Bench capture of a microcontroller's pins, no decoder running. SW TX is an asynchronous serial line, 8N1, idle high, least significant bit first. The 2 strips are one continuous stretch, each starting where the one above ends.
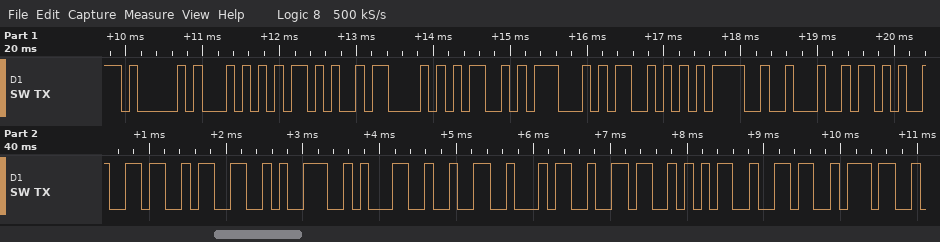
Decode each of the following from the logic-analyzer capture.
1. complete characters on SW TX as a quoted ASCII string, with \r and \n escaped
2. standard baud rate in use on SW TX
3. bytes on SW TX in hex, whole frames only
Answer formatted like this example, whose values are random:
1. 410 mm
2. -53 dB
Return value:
1. "AT+CMGS=\"+6391246567"
2. 9600 baud
3. 41 54 2B 43 4D 47 53 3D 22 2B 36 33 39 31 32 34 36 35 36 37
